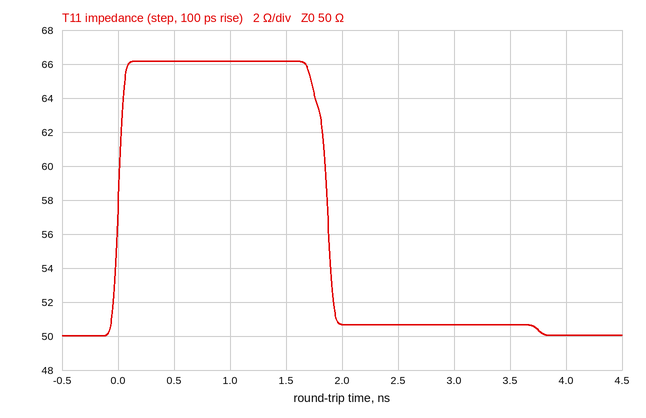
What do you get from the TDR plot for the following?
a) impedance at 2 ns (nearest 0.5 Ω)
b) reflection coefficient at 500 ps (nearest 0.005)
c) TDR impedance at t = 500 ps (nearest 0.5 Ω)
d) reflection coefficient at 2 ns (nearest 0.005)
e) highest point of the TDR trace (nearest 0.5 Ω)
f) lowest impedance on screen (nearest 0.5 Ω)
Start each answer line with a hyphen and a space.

- 50.5 Ω
- +0.140
- 66.0 Ω
- +0.005
- 66.0 Ω
- 50.0 Ω
